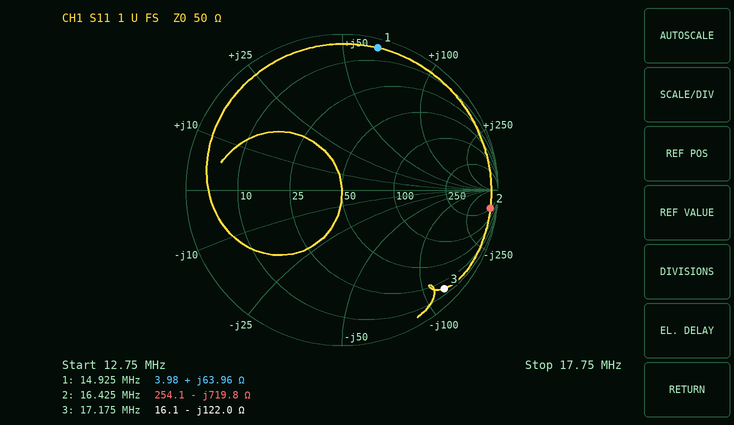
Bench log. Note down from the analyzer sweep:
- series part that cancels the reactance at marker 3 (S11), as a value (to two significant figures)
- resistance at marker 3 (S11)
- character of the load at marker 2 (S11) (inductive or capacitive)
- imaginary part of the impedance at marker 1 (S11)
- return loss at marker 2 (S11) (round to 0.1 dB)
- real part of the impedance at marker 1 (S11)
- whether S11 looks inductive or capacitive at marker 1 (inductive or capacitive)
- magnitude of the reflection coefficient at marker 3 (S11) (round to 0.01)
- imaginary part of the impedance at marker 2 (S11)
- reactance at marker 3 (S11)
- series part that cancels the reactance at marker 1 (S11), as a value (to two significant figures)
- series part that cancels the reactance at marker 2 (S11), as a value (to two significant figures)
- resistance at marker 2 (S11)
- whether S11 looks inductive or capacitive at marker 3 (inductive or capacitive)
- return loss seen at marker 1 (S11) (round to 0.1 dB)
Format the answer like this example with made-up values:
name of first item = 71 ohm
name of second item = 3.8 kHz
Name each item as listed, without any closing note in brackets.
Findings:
series part that cancels the reactance at marker 3 (S11), as a value = 1.1 µH
resistance at marker 3 = 16.1 Ω
character of the load at marker 2 (S11) = capacitive
imaginary part of the impedance at marker 1 = +63.96 Ω
return loss at marker 2 (S11) = 0.4 dB
real part of the impedance at marker 1 = 3.98 Ω
whether S11 looks inductive or capacitive at marker 1 = inductive
magnitude of the reflection coefficient at marker 3 (S11) = 0.91
imaginary part of the impedance at marker 2 = -719.8 Ω
reactance at marker 3 = -122.0 Ω
series part that cancels the reactance at marker 1 (S11), as a value = 170 pF
series part that cancels the reactance at marker 2 (S11), as a value = 7.0 µH
resistance at marker 2 = 254.1 Ω
whether S11 looks inductive or capacitive at marker 3 = capacitive
return loss seen at marker 1 (S11) = 0.5 dB
